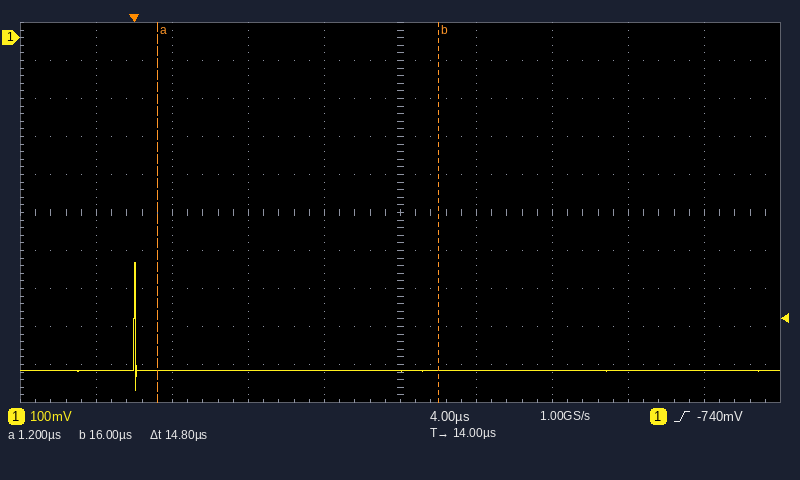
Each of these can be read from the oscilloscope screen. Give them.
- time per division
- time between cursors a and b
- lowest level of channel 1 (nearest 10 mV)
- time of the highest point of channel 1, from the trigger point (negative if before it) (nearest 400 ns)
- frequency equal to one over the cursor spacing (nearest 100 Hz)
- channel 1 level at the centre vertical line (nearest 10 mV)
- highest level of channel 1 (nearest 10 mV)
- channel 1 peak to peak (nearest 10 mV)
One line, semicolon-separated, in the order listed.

4 µs; 14.8 µs; -930 mV; 0.0 µs; 67.6 kHz; -880 mV; -590 mV; 340 mV
